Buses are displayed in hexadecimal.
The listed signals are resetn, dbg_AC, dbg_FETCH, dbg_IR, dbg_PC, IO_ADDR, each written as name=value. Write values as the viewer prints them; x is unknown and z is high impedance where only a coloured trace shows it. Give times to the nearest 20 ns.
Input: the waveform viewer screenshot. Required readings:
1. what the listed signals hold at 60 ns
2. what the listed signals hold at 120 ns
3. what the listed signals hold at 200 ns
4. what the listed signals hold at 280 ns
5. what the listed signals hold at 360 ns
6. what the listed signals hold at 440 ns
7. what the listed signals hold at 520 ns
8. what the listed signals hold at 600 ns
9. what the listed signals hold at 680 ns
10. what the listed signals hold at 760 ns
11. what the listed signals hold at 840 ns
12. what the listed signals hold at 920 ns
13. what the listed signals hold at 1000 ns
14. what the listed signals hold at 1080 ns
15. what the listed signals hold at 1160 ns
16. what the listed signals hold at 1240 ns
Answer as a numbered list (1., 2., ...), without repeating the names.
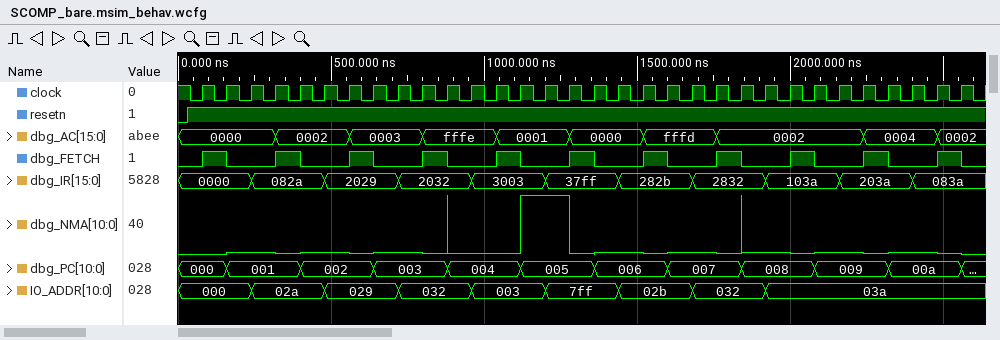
1. resetn=1, dbg_AC=0000, dbg_FETCH=0, dbg_IR=0000, dbg_PC=000, IO_ADDR=000
2. resetn=1, dbg_AC=0000, dbg_FETCH=1, dbg_IR=0000, dbg_PC=000, IO_ADDR=000
3. resetn=1, dbg_AC=0000, dbg_FETCH=0, dbg_IR=0000, dbg_PC=001, IO_ADDR=000
4. resetn=1, dbg_AC=0000, dbg_FETCH=0, dbg_IR=082a, dbg_PC=001, IO_ADDR=02a
5. resetn=1, dbg_AC=0002, dbg_FETCH=1, dbg_IR=082a, dbg_PC=001, IO_ADDR=02a
6. resetn=1, dbg_AC=0002, dbg_FETCH=0, dbg_IR=082a, dbg_PC=002, IO_ADDR=02a
7. resetn=1, dbg_AC=0002, dbg_FETCH=0, dbg_IR=2029, dbg_PC=002, IO_ADDR=029
8. resetn=1, dbg_AC=0003, dbg_FETCH=1, dbg_IR=2029, dbg_PC=002, IO_ADDR=029
9. resetn=1, dbg_AC=0003, dbg_FETCH=0, dbg_IR=2029, dbg_PC=003, IO_ADDR=029
10. resetn=1, dbg_AC=0003, dbg_FETCH=0, dbg_IR=2032, dbg_PC=003, IO_ADDR=032
11. resetn=1, dbg_AC=fffe, dbg_FETCH=1, dbg_IR=2032, dbg_PC=003, IO_ADDR=032
12. resetn=1, dbg_AC=fffe, dbg_FETCH=0, dbg_IR=2032, dbg_PC=004, IO_ADDR=032
13. resetn=1, dbg_AC=fffe, dbg_FETCH=0, dbg_IR=3003, dbg_PC=004, IO_ADDR=003
14. resetn=1, dbg_AC=0001, dbg_FETCH=1, dbg_IR=3003, dbg_PC=004, IO_ADDR=003
15. resetn=1, dbg_AC=0001, dbg_FETCH=0, dbg_IR=3003, dbg_PC=005, IO_ADDR=003
16. resetn=1, dbg_AC=0001, dbg_FETCH=0, dbg_IR=37ff, dbg_PC=005, IO_ADDR=7ff
